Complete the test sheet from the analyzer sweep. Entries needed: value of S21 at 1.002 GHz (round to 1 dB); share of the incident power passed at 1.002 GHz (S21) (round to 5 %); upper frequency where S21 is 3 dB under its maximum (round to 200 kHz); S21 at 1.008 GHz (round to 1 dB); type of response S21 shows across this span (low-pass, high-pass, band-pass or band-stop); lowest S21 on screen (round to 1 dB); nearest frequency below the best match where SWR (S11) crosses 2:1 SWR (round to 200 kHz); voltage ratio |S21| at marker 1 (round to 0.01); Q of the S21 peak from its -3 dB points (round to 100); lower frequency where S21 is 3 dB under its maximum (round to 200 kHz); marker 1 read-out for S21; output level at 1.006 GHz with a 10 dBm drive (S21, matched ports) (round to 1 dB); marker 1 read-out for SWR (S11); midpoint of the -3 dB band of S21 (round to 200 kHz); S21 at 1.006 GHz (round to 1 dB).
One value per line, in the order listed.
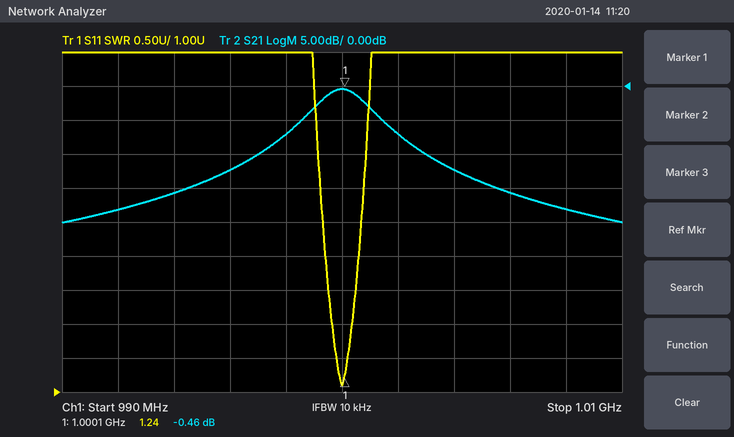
-7 dB
20 %
1.0010 GHz
-18 dB
band-pass
-20 dB
999.6 MHz
0.95
500
999.0 MHz
-0.46 dB
-6 dBm
1.24
1.0000 GHz
-16 dB
